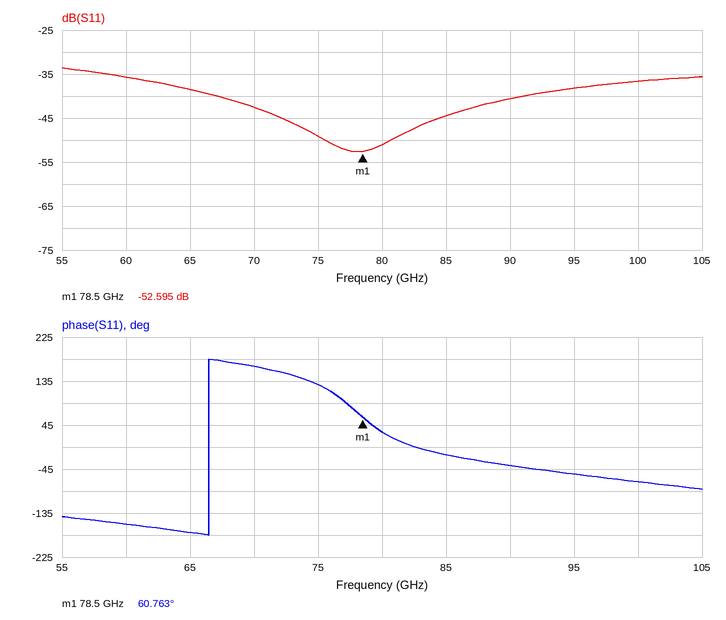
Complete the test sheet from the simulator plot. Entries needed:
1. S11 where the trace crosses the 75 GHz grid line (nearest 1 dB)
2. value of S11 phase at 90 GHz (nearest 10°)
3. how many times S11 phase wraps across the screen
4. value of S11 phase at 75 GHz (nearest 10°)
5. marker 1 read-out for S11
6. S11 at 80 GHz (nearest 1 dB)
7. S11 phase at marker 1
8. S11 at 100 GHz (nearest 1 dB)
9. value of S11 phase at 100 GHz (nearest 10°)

-49 dB
-40°
1
130°
-52.595 dB
-51 dB
60.763°
-37 dB
-70°
